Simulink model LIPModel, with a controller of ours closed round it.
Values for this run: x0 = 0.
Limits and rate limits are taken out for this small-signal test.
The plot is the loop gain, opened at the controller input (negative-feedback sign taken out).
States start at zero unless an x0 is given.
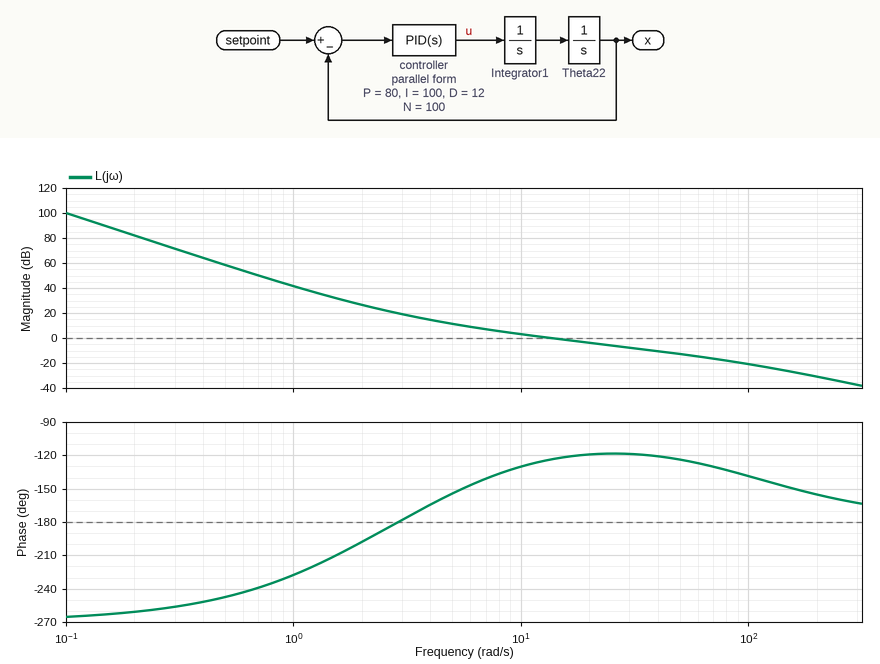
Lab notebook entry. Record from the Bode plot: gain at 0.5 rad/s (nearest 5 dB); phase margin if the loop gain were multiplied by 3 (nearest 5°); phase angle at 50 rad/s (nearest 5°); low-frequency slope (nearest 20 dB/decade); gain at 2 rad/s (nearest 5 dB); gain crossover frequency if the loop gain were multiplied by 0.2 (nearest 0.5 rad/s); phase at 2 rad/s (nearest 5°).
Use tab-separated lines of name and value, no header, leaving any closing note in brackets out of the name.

gain at 0.5 rad/s	60 dB
phase margin if the loop gain were multiplied by 3	60°
phase angle at 50 rad/s	-125°
low-frequency slope	-60 dB/decade
gain at 2 rad/s	25 dB
gain crossover frequency if the loop gain were multiplied by 0.2	4.0 rad/s
phase at 2 rad/s	-200°
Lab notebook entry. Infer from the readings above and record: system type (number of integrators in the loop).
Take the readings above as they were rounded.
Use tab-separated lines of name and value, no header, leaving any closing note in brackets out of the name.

system type	3
